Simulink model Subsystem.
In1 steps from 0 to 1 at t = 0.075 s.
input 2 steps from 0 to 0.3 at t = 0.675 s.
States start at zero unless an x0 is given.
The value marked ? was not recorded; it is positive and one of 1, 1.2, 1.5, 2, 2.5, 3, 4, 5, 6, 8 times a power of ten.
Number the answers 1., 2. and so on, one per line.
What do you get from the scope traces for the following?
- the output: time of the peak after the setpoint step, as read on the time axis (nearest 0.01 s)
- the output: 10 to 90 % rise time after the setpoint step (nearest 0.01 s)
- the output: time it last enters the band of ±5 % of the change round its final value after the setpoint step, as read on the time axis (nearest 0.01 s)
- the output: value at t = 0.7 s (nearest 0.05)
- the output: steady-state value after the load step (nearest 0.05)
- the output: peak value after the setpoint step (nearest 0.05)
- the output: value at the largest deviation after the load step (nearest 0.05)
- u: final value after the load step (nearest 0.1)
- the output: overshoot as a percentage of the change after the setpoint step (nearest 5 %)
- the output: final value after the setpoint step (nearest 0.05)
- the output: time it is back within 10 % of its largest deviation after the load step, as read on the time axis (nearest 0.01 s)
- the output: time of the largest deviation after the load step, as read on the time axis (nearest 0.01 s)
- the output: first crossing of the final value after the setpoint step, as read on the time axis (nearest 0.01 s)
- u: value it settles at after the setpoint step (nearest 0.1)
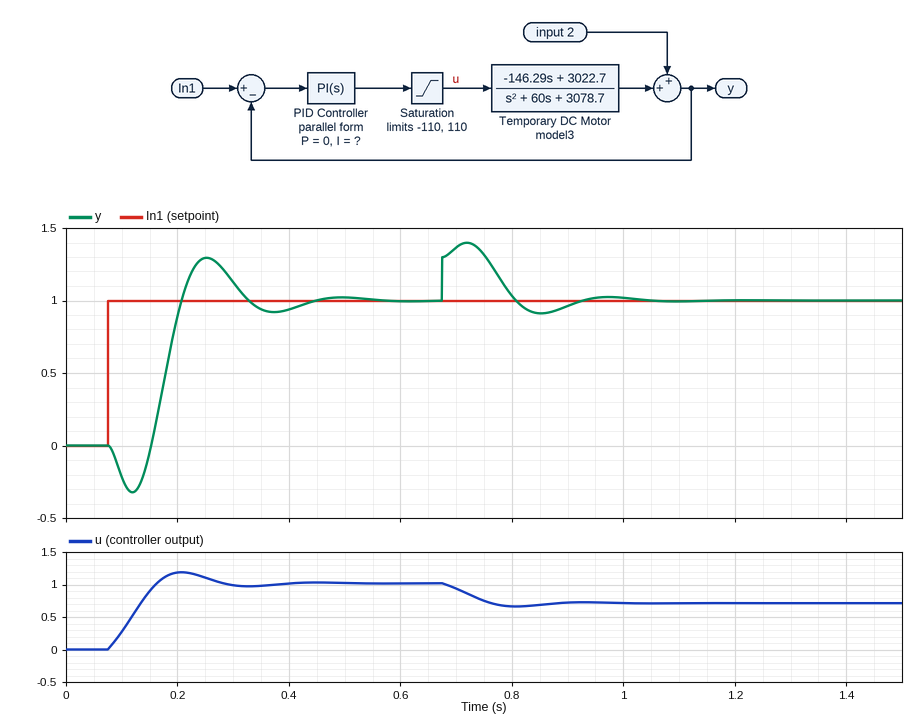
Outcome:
1. 0.25 s
2. 0.04 s
3. 0.41 s
4. 1.35
5. 1.00
6. 1.30
7. 1.40
8. 0.7
9. 30 %
10. 1.00
11. 0.90 s
12. 0.72 s
13. 0.21 s
14. 1.0
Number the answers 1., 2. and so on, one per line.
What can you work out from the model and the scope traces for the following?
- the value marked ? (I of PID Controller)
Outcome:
1. 10
